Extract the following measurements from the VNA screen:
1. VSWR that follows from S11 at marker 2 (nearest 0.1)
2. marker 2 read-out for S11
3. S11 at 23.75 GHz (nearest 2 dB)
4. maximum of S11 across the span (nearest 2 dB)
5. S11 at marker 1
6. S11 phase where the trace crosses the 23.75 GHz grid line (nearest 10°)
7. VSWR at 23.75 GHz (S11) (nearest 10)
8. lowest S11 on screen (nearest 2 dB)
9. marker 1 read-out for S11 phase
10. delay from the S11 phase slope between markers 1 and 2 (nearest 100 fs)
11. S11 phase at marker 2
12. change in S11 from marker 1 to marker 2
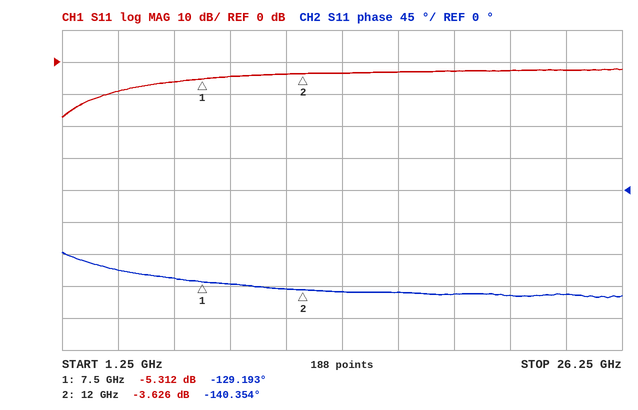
4.9
-3.626 dB
-2 dB
-2 dB
-5.312 dB
-150°
10
-18 dB
-129.193°
6.9 ps
-140.354°
1.686 dB
